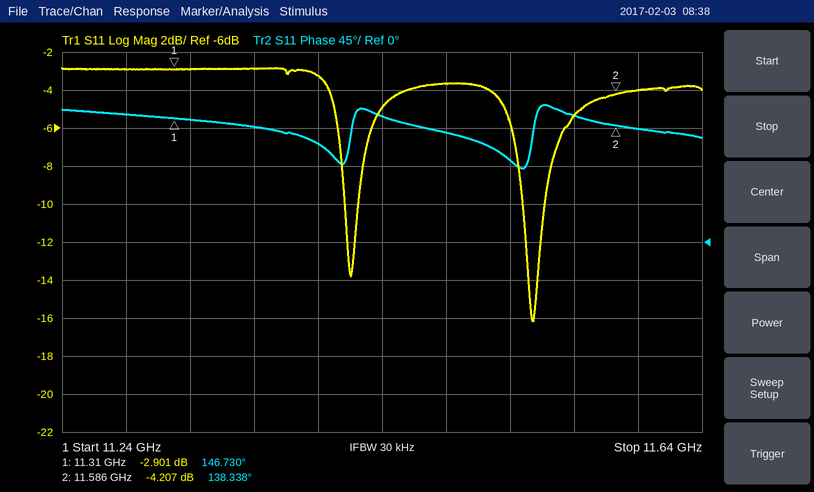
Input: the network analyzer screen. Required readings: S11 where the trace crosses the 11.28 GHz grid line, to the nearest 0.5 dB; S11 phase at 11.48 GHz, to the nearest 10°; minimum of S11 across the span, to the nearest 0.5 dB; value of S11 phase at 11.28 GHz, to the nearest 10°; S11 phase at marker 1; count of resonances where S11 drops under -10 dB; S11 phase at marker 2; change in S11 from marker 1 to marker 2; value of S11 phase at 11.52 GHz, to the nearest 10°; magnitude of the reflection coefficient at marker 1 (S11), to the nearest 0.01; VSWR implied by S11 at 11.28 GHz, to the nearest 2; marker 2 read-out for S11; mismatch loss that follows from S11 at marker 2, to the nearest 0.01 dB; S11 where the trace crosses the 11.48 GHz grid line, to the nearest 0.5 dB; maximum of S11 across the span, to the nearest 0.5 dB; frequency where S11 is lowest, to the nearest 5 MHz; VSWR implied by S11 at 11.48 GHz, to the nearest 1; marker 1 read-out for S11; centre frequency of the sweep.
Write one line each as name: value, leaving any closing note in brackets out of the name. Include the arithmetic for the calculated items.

S11 where the trace crosses the 11.28 GHz grid line, to the nearest 0.5 dB: -3.0 dB
S11 phase at 11.48 GHz, to the nearest 10°: 130°
minimum of S11 across the span, to the nearest 0.5 dB: -16.0 dB
value of S11 phase at 11.28 GHz, to the nearest 10°: 150°
S11 phase at marker 1: 146.730°
count of resonances where S11 drops under -10 dB: 2
S11 phase at marker 2: 138.338°
change in S11 from marker 1 to marker 2: -4.207 − (-2.901) = -1.306 dB
value of S11 phase at 11.52 GHz, to the nearest 10°: 100°
magnitude of the reflection coefficient at marker 1 (S11), to the nearest 0.01: 10^(-2.901/20) ≈ 0.72
VSWR implied by S11 at 11.28 GHz, to the nearest 2: |Γ| = 10^(-3/20) = 0.7079; VSWR = (1 + 0.7079)/(1 − 0.7079) ≈ 6
marker 2 read-out for S11: -4.207 dB
mismatch loss that follows from S11 at marker 2, to the nearest 0.01 dB: −10 log10(1 − 10^(-4.207/10)) ≈ 2.07 dB
S11 where the trace crosses the 11.48 GHz grid line, to the nearest 0.5 dB: -3.5 dB
maximum of S11 across the span, to the nearest 0.5 dB: -3.0 dB
frequency where S11 is lowest, to the nearest 5 MHz: 11.535 GHz
VSWR implied by S11 at 11.48 GHz, to the nearest 1: |Γ| = 10^(-3.5/20) = 0.6683; VSWR = (1 + 0.6683)/(1 − 0.6683) ≈ 5
marker 1 read-out for S11: -2.901 dB
centre frequency of the sweep: 11.44 GHz
